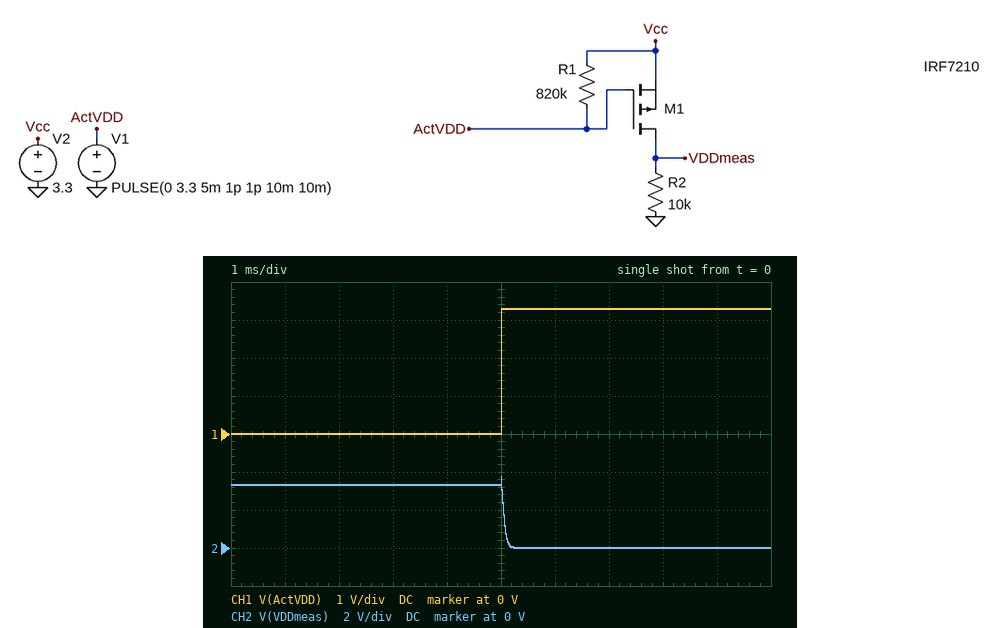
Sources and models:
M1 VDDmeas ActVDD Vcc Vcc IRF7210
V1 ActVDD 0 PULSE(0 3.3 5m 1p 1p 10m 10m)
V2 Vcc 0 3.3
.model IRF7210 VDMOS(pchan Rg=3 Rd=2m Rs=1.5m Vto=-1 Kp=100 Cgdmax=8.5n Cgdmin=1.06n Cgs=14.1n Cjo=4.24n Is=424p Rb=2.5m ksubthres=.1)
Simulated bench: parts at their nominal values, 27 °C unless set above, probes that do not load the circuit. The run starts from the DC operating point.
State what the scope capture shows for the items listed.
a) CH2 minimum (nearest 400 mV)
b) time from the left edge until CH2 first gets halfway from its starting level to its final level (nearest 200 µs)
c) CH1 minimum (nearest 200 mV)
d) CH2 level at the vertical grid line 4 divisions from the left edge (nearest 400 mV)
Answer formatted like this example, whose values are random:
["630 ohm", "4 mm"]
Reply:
["0 V", "5.0 ms", "0 V", "3.2 V"]
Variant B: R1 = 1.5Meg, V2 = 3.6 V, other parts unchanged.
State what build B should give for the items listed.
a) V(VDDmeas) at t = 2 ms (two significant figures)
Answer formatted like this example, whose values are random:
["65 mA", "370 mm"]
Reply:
["3.6 V"]
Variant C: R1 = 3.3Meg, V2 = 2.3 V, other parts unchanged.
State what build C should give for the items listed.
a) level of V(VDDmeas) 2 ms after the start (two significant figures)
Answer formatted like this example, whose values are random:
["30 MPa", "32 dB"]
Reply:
["2.3 V"]
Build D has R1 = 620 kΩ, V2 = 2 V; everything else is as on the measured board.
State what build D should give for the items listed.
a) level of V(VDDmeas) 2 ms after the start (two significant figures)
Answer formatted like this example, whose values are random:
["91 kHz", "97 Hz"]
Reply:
["2.0 V"]
